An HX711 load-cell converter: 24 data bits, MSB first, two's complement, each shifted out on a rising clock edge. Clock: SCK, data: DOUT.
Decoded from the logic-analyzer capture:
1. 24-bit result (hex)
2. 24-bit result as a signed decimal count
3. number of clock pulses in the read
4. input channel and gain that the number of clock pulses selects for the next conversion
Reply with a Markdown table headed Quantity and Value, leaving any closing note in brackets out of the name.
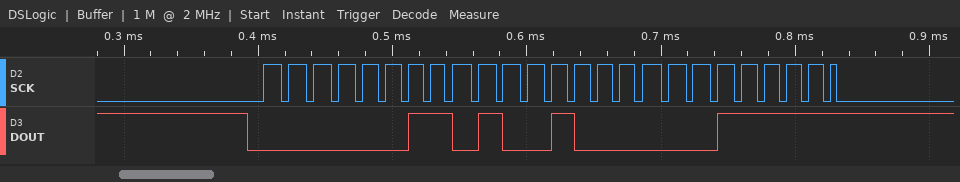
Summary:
| Quantity | Value |
|---|---|
| 24-bit result | 0x03481F |
| 24-bit result as a signed decimal count | 215071 |
| number of clock pulses in the read | 25 |
| input channel and gain that the number of clock pulses selects for the next conversion | channel A, gain 128 |
